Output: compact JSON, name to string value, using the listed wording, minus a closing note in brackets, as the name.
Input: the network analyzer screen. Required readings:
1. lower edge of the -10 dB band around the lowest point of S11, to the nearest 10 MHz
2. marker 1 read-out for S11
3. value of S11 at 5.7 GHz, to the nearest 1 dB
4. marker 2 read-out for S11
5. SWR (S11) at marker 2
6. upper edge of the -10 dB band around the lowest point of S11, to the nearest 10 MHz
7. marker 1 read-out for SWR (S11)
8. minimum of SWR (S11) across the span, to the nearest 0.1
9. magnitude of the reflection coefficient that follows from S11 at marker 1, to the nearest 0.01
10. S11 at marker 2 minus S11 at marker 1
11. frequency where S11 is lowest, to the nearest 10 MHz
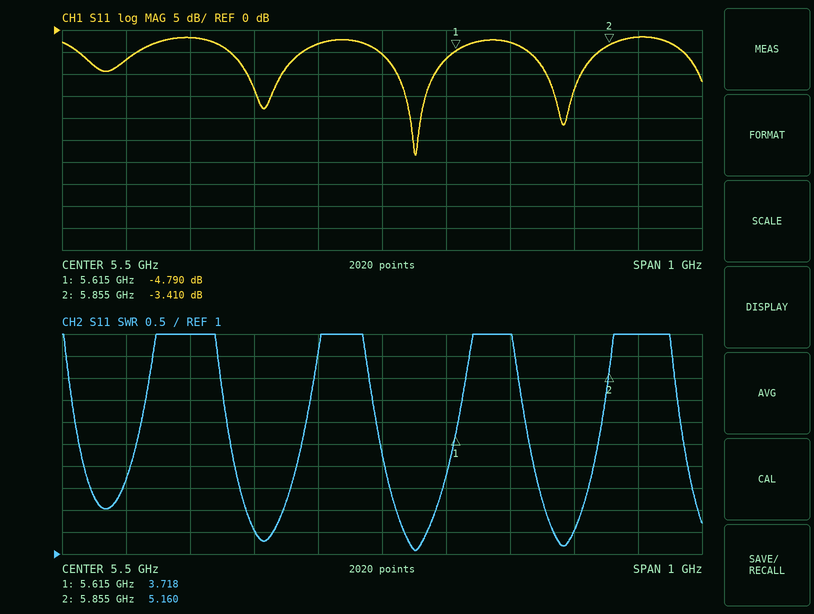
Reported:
{"lower edge of the -10 dB band around the lowest point of S11, to the nearest 10 MHz": "5.52 GHz", "marker 1 read-out for S11": "-4.790 dB", "value of S11 at 5.7 GHz, to the nearest 1 dB": "-3 dB", "marker 2 read-out for S11": "-3.410 dB", "SWR (S11) at marker 2": "5.160", "upper edge of the -10 dB band around the lowest point of S11, to the nearest 10 MHz": "5.58 GHz", "marker 1 read-out for SWR": "3.718", "minimum of SWR (S11) across the span, to the nearest 0.1": "1.1", "magnitude of the reflection coefficient that follows from S11 at marker 1, to the nearest 0.01": "0.58", "S11 at marker 2 minus S11 at marker 1": "1.380 dB", "frequency where S11 is lowest, to the nearest 10 MHz": "5.55 GHz"}
